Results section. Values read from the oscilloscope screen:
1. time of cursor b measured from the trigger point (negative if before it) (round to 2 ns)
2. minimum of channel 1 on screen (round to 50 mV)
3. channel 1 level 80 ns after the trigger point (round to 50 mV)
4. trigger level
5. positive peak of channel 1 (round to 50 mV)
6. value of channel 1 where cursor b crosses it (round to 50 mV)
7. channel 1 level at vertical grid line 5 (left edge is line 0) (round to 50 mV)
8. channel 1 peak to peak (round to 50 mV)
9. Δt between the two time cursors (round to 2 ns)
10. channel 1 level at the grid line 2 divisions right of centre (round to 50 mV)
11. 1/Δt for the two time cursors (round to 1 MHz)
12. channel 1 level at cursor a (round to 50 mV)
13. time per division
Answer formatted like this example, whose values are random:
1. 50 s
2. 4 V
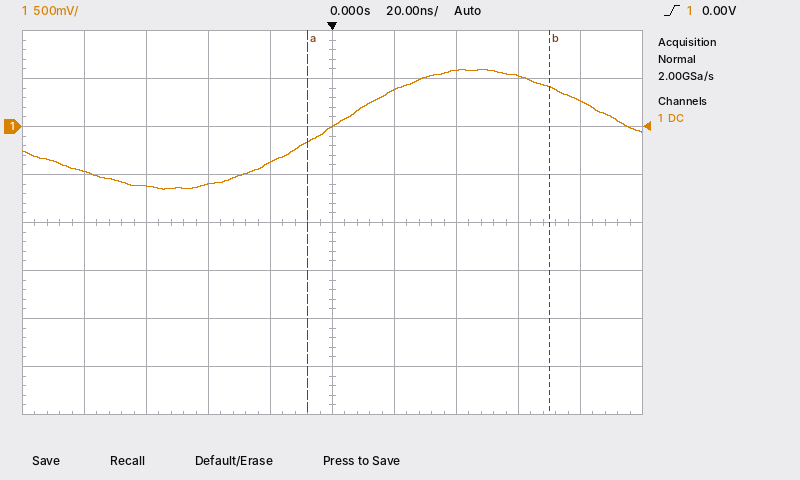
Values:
1. +70 ns
2. -650 mV
3. 250 mV
4. 0.00 V
5. 600 mV
6. 400 mV
7. 0 mV
8. 1.25 V
9. 78 ns
10. 600 mV
11. 13 MHz
12. -150 mV
13. 20 ns
